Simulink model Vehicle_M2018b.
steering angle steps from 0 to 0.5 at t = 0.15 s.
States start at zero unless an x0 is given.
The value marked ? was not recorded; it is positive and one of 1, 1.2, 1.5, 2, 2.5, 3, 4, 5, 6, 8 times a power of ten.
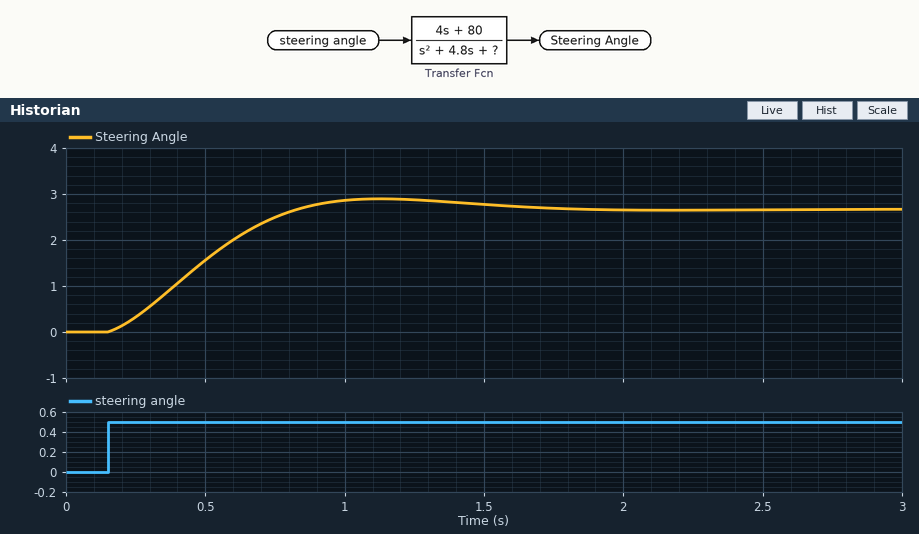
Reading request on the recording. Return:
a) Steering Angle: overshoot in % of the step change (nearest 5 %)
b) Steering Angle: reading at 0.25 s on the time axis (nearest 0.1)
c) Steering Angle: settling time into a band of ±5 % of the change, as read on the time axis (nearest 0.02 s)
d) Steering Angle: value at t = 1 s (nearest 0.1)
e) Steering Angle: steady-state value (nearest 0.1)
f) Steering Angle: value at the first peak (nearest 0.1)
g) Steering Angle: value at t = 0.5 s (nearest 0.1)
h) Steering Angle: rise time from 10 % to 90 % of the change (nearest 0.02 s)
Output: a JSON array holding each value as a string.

["10 %", "0.3", "1.44 s", "2.9", "2.7", "2.9", "1.6", "0.48 s"]
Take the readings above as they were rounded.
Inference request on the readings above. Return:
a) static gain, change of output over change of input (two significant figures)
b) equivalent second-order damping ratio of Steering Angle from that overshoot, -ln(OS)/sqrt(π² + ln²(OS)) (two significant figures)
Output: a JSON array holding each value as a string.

["5.4", "0.59"]
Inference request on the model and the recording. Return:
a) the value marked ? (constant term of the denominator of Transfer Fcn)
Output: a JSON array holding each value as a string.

["15"]
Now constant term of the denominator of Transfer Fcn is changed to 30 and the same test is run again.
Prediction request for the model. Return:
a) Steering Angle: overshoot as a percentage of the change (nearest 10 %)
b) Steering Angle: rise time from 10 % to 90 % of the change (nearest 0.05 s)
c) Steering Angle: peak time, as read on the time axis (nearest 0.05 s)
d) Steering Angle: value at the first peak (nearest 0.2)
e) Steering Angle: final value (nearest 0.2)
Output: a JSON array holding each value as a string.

["20 %", "0.25 s", "0.75 s", "1.6", "1.4"]
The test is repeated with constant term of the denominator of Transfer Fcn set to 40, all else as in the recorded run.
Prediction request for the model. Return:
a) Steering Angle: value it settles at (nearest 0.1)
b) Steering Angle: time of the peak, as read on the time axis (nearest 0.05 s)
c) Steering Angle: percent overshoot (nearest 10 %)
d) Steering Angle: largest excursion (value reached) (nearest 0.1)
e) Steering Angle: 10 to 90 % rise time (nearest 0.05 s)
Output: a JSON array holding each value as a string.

["1.0", "0.65 s", "30 %", "1.3", "0.20 s"]
